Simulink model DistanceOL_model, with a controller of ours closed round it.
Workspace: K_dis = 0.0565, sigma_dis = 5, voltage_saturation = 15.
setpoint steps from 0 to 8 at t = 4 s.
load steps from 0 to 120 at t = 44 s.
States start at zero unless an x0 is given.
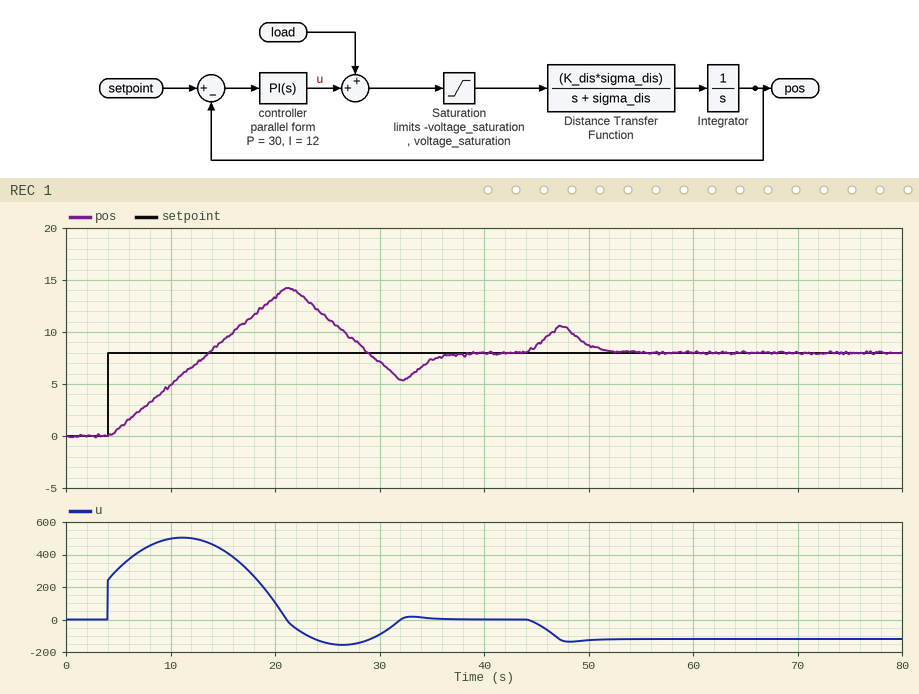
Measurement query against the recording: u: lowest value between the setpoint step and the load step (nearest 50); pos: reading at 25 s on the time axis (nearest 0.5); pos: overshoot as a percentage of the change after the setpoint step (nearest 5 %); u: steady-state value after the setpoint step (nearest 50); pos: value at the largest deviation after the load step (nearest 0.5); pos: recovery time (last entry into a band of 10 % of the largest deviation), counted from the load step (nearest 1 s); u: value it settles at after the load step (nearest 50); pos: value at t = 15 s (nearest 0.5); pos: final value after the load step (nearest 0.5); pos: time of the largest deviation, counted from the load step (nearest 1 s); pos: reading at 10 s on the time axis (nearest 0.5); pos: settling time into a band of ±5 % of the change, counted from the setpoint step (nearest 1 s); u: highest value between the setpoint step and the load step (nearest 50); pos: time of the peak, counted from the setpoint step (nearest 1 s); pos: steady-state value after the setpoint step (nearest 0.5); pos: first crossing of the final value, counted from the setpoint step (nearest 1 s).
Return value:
-150
11.5
80 %
0
10.5
8 s
-100
9.0
8.0
3 s
5.0
32 s
500
17 s
8.0
10 s
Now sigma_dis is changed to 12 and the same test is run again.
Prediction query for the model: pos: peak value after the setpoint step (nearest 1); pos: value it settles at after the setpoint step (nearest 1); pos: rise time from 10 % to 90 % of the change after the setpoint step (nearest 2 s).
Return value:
14
8
8 s
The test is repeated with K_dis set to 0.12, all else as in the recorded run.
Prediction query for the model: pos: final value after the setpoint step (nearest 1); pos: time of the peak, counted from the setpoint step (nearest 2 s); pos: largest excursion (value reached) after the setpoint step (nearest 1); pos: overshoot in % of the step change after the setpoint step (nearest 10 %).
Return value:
8
8 s
13
60 %
